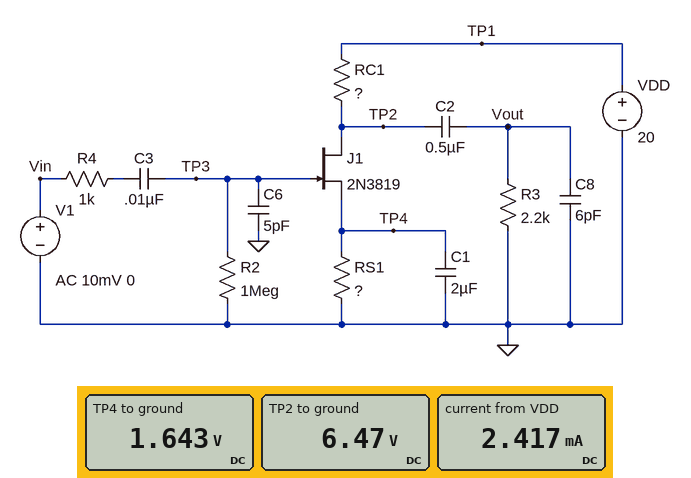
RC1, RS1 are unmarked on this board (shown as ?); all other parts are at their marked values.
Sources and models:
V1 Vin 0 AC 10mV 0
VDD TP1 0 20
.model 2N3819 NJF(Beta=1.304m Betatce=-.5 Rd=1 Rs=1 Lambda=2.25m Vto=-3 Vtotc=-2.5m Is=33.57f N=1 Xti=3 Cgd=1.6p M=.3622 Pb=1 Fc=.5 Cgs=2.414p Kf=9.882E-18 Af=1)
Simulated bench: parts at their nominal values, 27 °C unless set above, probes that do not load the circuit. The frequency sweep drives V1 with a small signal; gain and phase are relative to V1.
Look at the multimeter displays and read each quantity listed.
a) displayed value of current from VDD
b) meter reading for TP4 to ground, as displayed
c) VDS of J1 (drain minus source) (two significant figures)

2.417 mA
1.643 V
4.8 V
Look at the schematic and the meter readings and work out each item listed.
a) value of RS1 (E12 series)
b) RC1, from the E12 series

680 Ω
5.6 kΩ
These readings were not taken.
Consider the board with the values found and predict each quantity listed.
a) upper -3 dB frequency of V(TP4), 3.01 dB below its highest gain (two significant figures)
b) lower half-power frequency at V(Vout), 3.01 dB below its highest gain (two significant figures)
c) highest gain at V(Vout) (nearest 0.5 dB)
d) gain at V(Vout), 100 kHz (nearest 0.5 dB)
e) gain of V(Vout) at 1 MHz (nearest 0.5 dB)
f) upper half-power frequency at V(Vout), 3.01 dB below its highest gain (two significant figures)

430 Hz
370 Hz
15.0 dB
15.0 dB
15.0 dB
9.2 MHz
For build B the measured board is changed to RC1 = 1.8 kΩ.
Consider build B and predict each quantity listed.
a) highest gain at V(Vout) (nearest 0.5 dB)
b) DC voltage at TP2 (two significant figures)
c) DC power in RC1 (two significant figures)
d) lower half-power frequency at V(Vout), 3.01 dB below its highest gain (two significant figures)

11.0 dB
16 V
11 mW
390 Hz
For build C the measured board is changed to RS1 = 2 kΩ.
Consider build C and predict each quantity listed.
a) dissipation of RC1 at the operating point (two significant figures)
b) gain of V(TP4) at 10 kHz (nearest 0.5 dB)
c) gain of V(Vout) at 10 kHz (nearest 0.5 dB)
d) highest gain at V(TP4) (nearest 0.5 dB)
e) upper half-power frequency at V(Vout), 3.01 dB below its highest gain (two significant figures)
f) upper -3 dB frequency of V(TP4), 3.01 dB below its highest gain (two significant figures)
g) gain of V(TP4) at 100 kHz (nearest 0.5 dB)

6.2 mW
-34.5 dB
11.5 dB
-2.5 dB
11 MHz
260 Hz
-54.5 dB
